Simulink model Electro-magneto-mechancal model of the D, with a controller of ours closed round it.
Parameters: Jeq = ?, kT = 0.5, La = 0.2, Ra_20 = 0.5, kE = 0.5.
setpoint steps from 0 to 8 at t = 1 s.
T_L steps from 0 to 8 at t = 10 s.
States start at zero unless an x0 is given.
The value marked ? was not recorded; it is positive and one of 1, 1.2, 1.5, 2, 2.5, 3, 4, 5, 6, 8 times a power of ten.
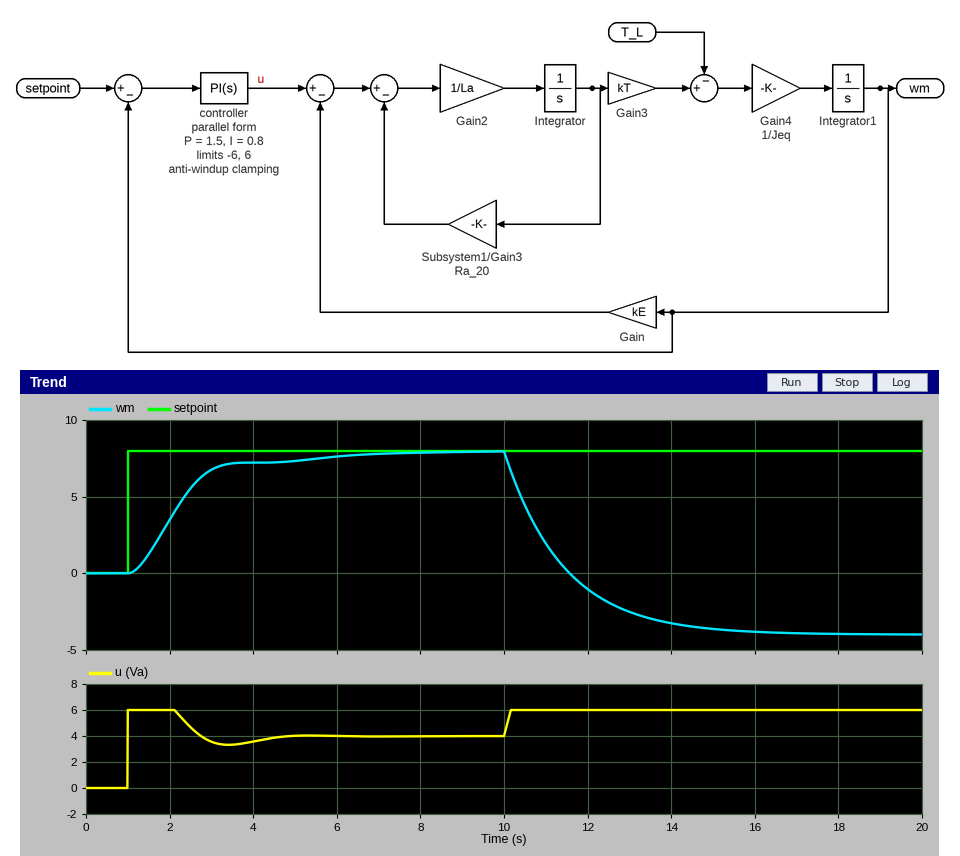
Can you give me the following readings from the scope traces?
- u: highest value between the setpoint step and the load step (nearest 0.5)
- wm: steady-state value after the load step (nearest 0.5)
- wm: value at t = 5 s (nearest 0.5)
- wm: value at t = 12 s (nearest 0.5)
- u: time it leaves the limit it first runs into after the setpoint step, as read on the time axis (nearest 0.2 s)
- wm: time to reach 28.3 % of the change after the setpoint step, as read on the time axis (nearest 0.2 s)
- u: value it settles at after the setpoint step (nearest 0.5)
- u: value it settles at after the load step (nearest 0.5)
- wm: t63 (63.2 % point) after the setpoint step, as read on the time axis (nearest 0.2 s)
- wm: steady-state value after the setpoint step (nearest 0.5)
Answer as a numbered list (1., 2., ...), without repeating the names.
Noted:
1. 6.0
2. -4.0
3. 7.5
4. -1.0
5. 2.2 s
6. 1.8 s
7. 4.0
8. 6.0
9. 2.4 s
10. 8.0
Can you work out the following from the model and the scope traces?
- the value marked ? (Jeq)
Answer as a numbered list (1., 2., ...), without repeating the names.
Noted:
1. 1
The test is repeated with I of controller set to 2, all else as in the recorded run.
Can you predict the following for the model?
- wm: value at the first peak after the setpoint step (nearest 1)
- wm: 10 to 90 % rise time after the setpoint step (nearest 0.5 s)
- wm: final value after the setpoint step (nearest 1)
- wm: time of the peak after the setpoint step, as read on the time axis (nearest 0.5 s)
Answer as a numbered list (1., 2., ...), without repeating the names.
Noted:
1. 8
2. 1.5 s
3. 8
4. 4.0 s
